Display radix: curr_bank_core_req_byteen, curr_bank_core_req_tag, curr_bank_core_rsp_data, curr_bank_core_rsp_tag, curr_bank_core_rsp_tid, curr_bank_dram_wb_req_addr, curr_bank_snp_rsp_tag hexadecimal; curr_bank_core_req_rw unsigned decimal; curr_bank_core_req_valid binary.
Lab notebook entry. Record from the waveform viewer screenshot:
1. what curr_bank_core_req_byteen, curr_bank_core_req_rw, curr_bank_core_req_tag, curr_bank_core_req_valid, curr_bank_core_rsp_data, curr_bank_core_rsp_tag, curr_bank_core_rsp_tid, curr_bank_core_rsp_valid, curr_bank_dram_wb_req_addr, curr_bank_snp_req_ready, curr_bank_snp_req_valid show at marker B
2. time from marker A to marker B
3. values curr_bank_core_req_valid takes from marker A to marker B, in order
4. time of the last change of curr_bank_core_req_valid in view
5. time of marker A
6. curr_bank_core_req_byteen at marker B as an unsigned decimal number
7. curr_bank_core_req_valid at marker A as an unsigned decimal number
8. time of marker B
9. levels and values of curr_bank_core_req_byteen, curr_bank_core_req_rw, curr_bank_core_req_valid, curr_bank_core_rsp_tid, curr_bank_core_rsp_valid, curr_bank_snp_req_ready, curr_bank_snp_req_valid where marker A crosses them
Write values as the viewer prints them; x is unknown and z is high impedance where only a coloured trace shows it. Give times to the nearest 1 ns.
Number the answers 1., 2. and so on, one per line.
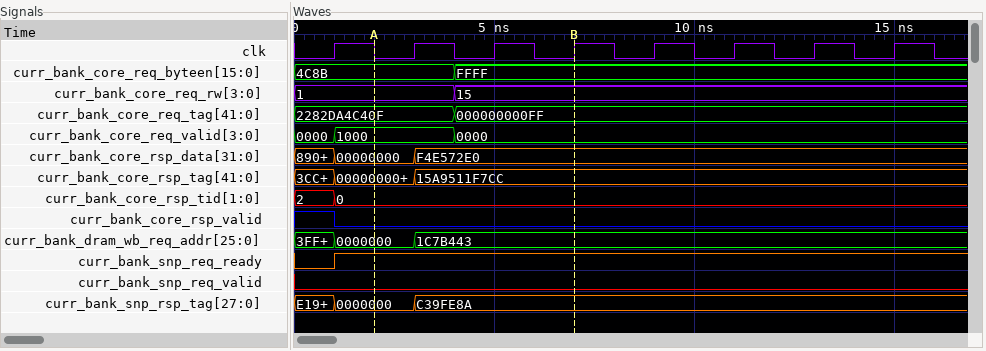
1. curr_bank_core_req_byteen=FFFF, curr_bank_core_req_rw=15, curr_bank_core_req_tag=000000000FF, curr_bank_core_req_valid=0000, curr_bank_core_rsp_data=F4E572E0, curr_bank_core_rsp_tag=15A9511F7CC, curr_bank_core_rsp_tid=0, curr_bank_core_rsp_valid=0, curr_bank_dram_wb_req_addr=1C7B443, curr_bank_snp_req_ready=1, curr_bank_snp_req_valid=0
2. 5 ns
3. 1000, 0000
4. 4 ns
5. 2 ns
6. 65535
7. 8
8. 7 ns
9. curr_bank_core_req_byteen=4C8B, curr_bank_core_req_rw=1, curr_bank_core_req_valid=1000, curr_bank_core_rsp_tid=0, curr_bank_core_rsp_valid=0, curr_bank_snp_req_ready=1, curr_bank_snp_req_valid=0
